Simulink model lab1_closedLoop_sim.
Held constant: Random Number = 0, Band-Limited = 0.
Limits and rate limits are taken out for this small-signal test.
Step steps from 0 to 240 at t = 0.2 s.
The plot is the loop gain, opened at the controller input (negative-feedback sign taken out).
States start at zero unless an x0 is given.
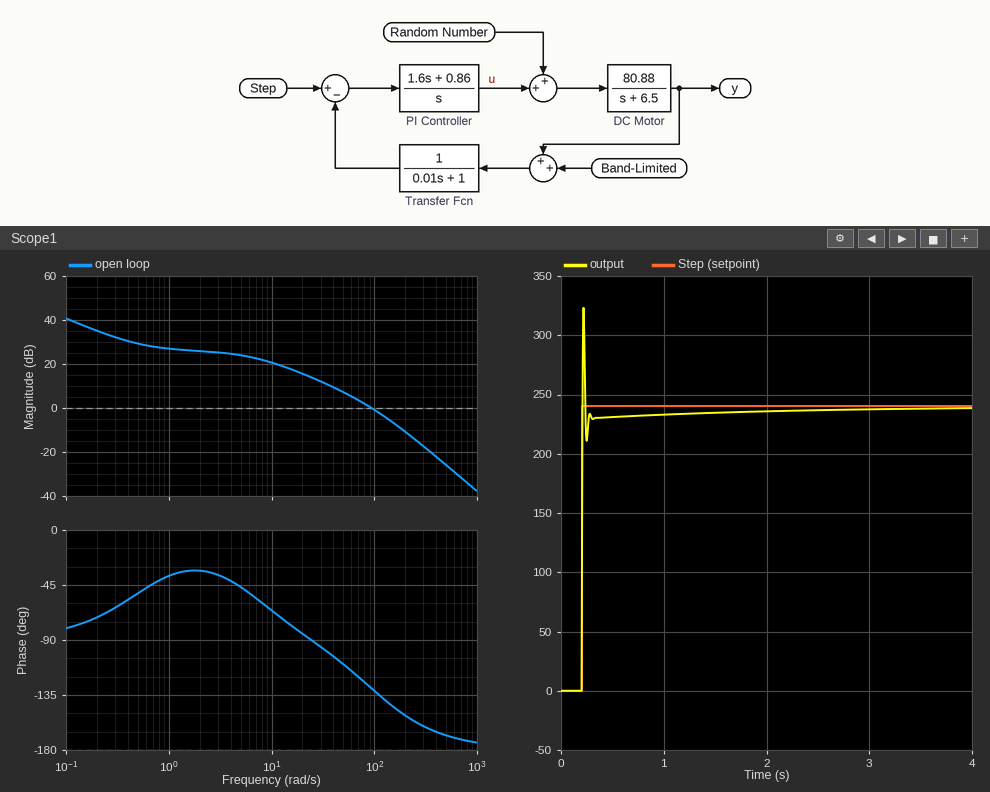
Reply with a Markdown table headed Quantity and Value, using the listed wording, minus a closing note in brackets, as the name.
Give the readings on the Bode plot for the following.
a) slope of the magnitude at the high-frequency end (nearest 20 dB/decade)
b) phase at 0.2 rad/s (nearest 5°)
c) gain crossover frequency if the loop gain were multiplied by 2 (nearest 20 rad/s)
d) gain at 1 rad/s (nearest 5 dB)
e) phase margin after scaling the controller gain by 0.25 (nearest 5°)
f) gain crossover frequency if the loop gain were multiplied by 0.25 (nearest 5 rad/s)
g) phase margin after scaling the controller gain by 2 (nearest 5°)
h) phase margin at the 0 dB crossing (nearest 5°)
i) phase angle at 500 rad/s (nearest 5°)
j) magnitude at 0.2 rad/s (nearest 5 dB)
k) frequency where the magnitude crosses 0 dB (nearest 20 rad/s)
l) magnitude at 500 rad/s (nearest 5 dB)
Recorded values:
| Quantity | Value |
|---|---|
| slope of the magnitude at the high-frequency end | -40 dB/decade |
| phase at 0.2 rad/s | -70° |
| gain crossover frequency if the loop gain were multiplied by 2 | 140 rad/s |
| gain at 1 rad/s | 25 dB |
| phase margin after scaling the controller gain by 0.25 | 85° |
| gain crossover frequency if the loop gain were multiplied by 0.25 | 30 rad/s |
| phase margin after scaling the controller gain by 2 | 35° |
| phase margin at the 0 dB crossing | 50° |
| phase angle at 500 rad/s | -170° |
| magnitude at 0.2 rad/s | 35 dB |
| frequency where the magnitude crosses 0 dB | 100 rad/s |
| magnitude at 500 rad/s | -25 dB |
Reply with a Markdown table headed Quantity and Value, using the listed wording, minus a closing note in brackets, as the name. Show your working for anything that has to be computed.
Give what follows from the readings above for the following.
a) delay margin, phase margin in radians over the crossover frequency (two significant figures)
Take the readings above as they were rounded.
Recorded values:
| Quantity | Value |
|---|---|
| delay margin, phase margin in radians over the crossover frequency | 50 × π / 180 / 100 = 0.0087 s |
